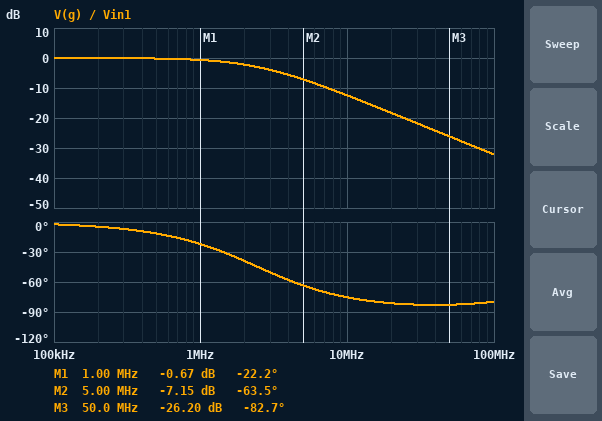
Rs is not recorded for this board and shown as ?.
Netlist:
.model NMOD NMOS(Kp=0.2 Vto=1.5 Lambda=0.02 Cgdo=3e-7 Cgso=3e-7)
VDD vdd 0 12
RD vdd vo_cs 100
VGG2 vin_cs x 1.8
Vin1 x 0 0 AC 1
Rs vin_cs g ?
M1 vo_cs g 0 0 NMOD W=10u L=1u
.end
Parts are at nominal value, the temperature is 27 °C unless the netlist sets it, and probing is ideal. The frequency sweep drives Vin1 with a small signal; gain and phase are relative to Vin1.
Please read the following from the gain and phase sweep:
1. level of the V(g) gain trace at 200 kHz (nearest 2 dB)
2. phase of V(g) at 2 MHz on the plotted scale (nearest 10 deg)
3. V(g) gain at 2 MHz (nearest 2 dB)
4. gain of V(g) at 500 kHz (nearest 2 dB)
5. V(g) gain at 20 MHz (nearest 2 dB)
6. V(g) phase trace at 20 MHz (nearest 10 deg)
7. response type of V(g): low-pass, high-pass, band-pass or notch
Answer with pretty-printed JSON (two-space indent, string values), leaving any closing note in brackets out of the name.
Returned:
{
  "level of the V(g) gain trace at 200 kHz": "0 dB",
  "phase of V(g) at 2 MHz on the plotted scale": "-40 deg",
  "V(g) gain at 2 MHz": "-2 dB",
  "gain of V(g) at 500 kHz": "0 dB",
  "V(g) gain at 20 MHz": "-18 dB",
  "V(g) phase trace at 20 MHz": "-80 deg",
  "response type of V(g): low-pass, high-pass, band-pass or notch": "low-pass"
}
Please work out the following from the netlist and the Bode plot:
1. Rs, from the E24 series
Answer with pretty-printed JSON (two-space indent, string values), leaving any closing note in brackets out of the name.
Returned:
{
  "Rs, from the E24 series": "390 Ω"
}
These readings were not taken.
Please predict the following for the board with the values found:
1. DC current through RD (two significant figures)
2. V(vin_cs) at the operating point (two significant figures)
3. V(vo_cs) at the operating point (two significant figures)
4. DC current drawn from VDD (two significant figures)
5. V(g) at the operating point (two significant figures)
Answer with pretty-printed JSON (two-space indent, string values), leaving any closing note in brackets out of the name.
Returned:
{
  "DC current through RD": "95 mA",
  "V(vin_cs) at the operating point": "1.8 V",
  "V(vo_cs) at the operating point": "2.5 V",
  "DC current drawn from VDD": "95 mA",
  "V(g) at the operating point": "1.8 V"
}
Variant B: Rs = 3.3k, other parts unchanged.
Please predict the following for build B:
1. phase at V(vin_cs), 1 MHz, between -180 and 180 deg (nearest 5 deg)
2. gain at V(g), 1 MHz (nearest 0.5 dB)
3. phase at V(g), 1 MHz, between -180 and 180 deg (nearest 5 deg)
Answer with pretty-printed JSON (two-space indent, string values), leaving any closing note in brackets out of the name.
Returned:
{
  "phase at V(vin_cs), 1 MHz, between -180 and 180 deg": "0 deg",
  "gain at V(g), 1 MHz": "-11.0 dB",
  "phase at V(g), 1 MHz, between -180 and 180 deg": "-75 deg"
}
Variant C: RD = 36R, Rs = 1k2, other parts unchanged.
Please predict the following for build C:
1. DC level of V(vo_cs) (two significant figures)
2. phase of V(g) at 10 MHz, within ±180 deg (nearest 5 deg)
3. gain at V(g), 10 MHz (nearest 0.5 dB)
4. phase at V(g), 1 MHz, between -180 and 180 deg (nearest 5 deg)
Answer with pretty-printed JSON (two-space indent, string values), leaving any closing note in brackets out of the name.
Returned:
{
  "DC level of V(vo_cs)": "8.2 V",
  "phase of V(g) at 10 MHz, within ±180 deg": "-80 deg",
  "gain at V(g), 10 MHz": "-15.5 dB",
  "phase at V(g), 1 MHz, between -180 and 180 deg": "-30 deg"
}
